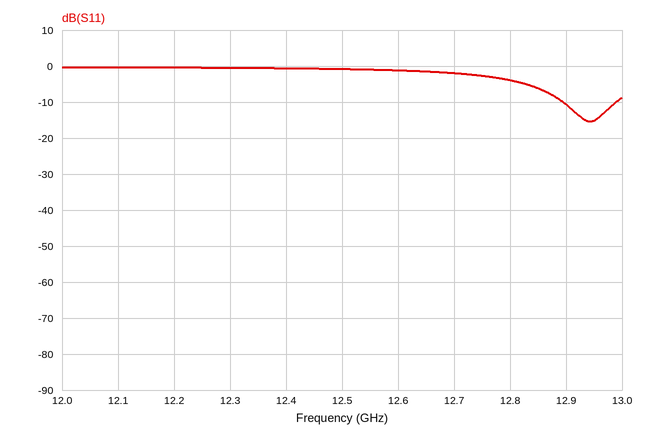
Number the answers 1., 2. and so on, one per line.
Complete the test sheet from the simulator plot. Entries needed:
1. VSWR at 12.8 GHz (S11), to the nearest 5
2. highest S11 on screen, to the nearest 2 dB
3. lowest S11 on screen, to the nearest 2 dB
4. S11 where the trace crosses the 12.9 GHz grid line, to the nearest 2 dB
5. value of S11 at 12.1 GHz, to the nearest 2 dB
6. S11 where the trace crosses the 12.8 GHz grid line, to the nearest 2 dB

1. 5
2. 0 dB
3. -16 dB
4. -10 dB
5. 0 dB
6. -4 dB
